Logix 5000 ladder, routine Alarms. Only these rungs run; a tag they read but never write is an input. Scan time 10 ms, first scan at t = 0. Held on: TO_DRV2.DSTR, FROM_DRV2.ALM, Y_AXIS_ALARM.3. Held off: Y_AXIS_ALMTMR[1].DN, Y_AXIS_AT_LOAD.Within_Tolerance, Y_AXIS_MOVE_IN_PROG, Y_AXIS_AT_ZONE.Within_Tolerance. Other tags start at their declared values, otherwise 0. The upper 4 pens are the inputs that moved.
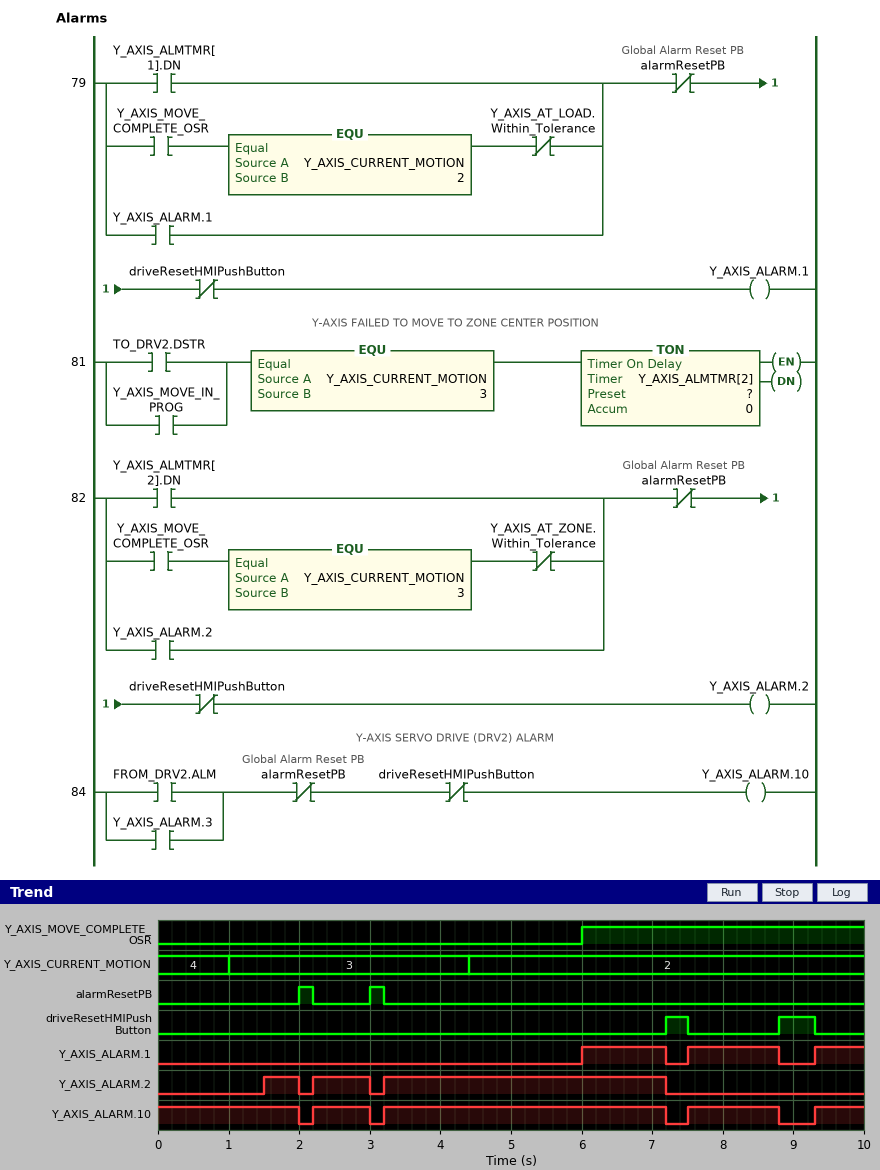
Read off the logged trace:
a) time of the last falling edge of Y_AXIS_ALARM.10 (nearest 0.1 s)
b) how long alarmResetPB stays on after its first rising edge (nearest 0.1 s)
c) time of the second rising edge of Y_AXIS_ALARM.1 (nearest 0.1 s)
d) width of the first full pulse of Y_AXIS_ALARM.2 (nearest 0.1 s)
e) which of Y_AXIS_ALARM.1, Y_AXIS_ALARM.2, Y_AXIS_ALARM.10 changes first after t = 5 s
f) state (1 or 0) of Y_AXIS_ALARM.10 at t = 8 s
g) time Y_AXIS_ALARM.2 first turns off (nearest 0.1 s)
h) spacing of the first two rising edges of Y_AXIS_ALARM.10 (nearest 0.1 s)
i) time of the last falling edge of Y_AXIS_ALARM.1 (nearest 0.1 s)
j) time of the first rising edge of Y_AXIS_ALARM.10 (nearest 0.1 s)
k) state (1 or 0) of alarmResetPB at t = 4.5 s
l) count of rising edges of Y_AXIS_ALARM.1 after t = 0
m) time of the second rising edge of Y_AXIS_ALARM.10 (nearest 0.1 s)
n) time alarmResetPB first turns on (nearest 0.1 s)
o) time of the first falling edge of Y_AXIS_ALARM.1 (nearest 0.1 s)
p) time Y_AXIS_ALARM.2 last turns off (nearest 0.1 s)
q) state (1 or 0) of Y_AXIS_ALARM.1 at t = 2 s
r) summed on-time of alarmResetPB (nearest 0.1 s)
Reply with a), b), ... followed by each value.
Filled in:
a) 8.8 s
b) 0.2 s
c) 7.5 s
d) 0.5 s
e) Y_AXIS_ALARM.1
f) 1
g) 2.0 s
h) 1.0 s
i) 8.8 s
j) 2.2 s
k) 0
l) 3
m) 3.2 s
n) 2.0 s
o) 7.2 s
p) 7.2 s
q) 0
r) 0.4 s
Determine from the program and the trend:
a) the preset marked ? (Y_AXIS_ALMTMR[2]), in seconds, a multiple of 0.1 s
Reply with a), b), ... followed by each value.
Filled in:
a) 0.5 s
